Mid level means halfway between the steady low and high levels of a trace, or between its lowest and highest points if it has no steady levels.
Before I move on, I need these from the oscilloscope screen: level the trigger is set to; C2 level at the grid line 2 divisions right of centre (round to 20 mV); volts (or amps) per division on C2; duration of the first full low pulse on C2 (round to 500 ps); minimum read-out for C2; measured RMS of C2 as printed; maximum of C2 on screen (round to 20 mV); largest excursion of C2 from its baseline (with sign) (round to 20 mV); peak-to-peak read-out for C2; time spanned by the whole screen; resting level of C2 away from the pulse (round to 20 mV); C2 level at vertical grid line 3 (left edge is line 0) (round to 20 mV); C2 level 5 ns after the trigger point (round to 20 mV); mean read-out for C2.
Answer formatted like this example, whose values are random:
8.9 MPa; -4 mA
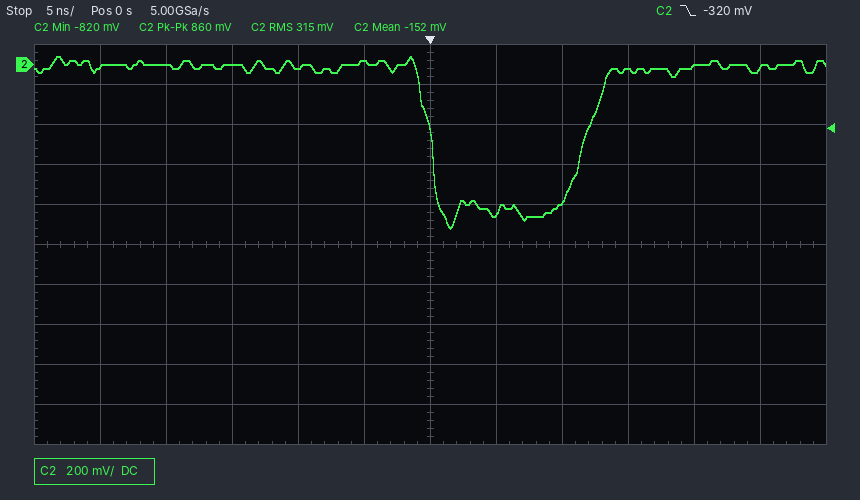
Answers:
-320 mV; -680 mV; 200 mV; 11.5 ns; -820 mV; 315 mV; 40 mV; -800 mV; 860 mV; 60 ns; -20 mV; 0 mV; -740 mV; -152 mV
